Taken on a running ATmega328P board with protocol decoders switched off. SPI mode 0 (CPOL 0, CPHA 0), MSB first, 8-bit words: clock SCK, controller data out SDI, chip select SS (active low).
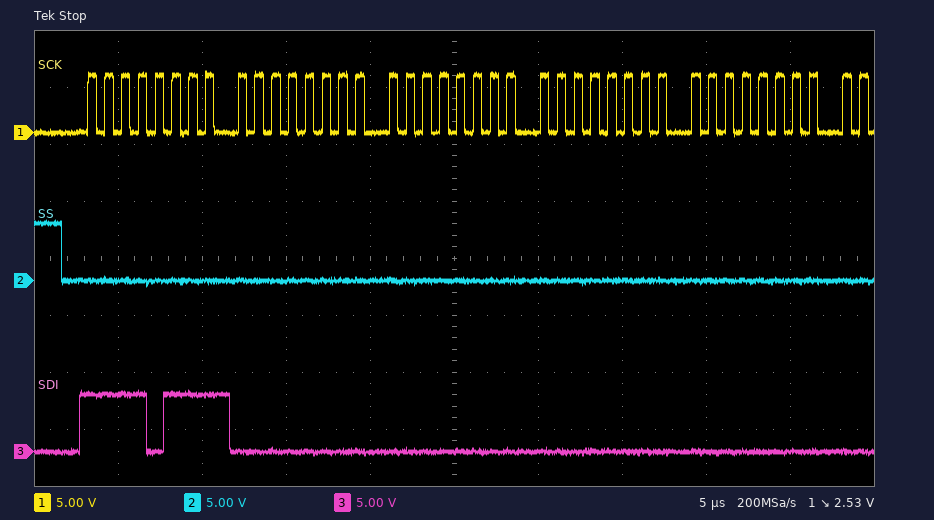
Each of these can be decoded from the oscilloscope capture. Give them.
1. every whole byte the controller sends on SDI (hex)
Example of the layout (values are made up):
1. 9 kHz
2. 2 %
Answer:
1. F7 00 00 00 00
